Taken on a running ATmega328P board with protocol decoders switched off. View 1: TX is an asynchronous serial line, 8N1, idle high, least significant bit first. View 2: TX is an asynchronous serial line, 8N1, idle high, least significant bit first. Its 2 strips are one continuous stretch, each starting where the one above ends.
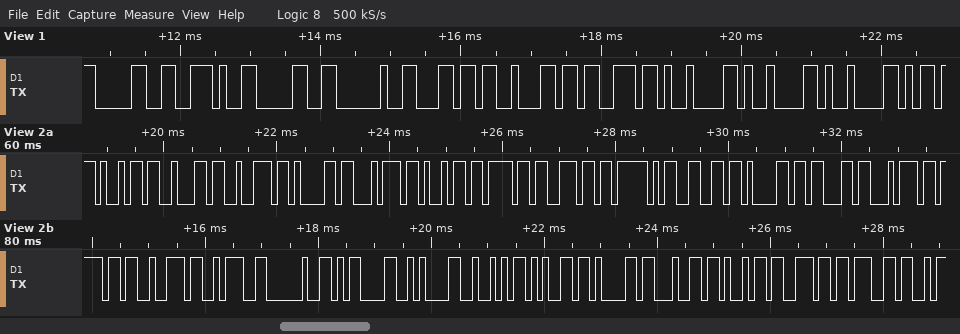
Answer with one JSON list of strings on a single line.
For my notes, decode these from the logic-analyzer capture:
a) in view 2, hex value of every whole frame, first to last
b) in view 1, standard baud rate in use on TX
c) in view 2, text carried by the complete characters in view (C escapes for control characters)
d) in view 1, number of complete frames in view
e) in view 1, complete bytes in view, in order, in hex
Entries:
["0x69 0x62 0x72 0x61 0x74 0x69 0x6F 0x6E 0x5F 0x66 0x61 0x63 0x74 0x6F 0x72 0x3A 0x20 0x0D 0x0A 0x52 0x65 0x61 0x64 0x69 0x6E 0x67", "9600 baud", "\"ibration_factor: \\r\\nReading\"", "10", "0x30 0x2E 0x30 0x20 0x6C 0x62 0x73 0x09 0x09 0x09"]
